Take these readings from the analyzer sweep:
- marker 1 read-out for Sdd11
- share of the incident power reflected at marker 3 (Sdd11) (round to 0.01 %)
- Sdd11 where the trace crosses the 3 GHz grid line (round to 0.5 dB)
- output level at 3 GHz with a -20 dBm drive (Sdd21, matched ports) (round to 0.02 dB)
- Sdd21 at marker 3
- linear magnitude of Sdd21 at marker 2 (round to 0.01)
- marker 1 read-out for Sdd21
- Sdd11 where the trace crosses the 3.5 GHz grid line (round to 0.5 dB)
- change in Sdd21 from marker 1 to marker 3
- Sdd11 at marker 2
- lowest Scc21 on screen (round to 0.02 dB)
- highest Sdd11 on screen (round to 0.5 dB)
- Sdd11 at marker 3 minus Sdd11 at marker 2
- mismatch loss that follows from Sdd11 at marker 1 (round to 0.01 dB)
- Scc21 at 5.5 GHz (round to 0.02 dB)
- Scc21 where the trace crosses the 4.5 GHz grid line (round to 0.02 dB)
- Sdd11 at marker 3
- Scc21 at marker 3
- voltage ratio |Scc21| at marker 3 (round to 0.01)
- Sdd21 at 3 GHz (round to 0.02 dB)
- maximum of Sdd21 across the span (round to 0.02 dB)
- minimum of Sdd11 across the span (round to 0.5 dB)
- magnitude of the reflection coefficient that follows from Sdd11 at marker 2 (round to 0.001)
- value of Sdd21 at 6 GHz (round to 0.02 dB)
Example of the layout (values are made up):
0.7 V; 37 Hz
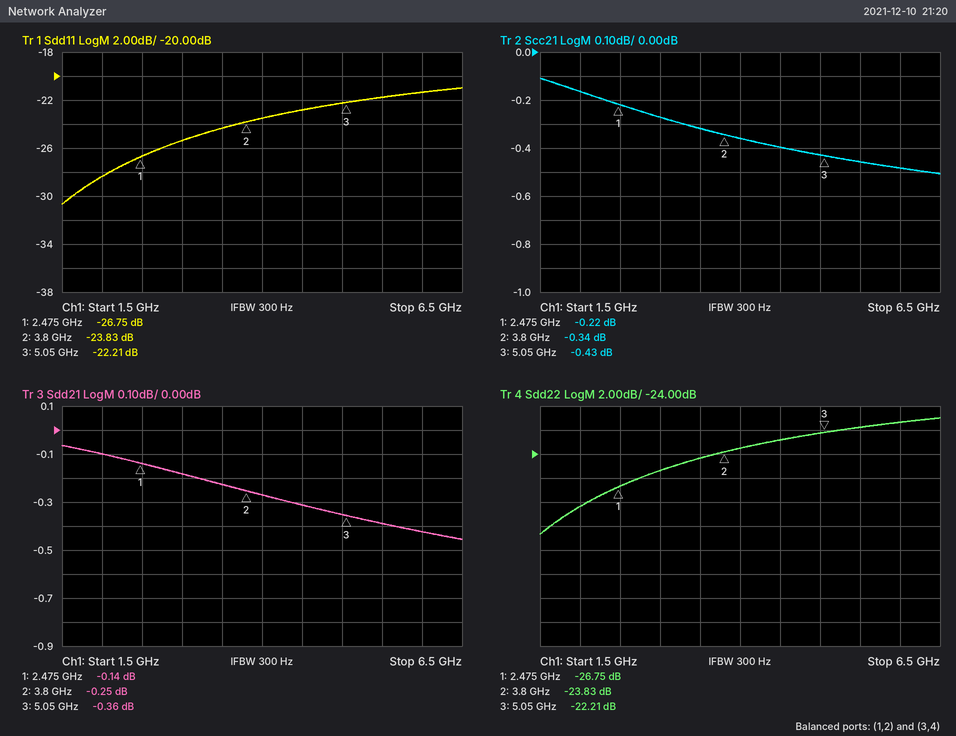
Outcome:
-26.75 dB; 0.60 %; -25.5 dB; -20.18 dBm; -0.36 dB; 0.97; -0.14 dB; -24.5 dB; -0.22 dB; -23.83 dB; -0.50 dB; -21.0 dB; 1.62 dB; 0.01 dB; -0.46 dB; -0.40 dB; -22.21 dB; -0.43 dB; 0.95; -0.18 dB; -0.06 dB; -30.5 dB; 0.064; -0.42 dB
